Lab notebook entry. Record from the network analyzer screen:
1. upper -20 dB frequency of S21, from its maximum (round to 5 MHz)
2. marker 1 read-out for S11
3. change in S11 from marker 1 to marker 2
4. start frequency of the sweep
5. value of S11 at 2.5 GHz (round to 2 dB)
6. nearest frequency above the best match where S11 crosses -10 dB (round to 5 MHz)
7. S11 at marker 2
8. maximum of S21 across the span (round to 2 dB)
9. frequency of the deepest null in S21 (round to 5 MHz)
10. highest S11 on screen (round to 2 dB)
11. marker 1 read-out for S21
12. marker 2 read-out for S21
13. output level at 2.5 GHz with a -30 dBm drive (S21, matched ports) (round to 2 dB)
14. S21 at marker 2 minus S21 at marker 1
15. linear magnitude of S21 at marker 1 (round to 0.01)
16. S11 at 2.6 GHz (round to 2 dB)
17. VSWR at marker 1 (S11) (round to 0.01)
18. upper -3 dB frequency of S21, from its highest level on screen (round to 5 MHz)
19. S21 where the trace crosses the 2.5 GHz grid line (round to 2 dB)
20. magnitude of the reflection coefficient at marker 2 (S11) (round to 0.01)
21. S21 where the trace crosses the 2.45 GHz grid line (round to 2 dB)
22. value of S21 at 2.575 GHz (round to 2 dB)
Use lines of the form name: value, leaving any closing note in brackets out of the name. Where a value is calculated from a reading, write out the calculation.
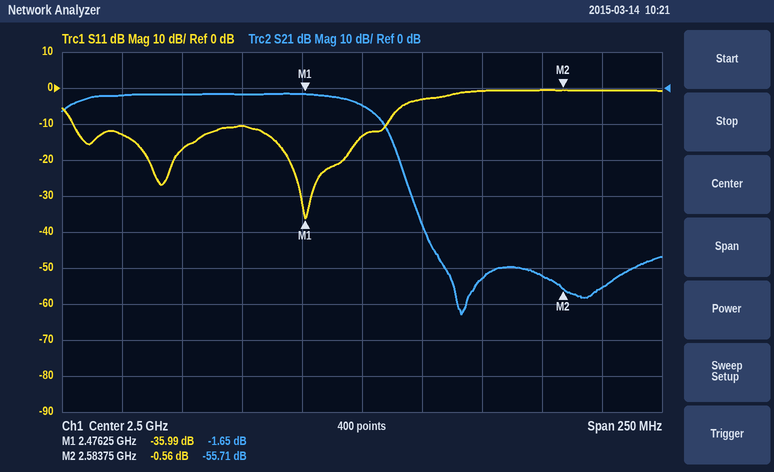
upper -20 dB frequency of S21, from its maximum: 2.515 GHz
marker 1 read-out for S11: -35.99 dB
change in S11 from marker 1 to marker 2: -0.56 − (-35.99) = 35.43 dB
start frequency of the sweep: 2.375 GHz
value of S11 at 2.5 GHz: -14 dB
nearest frequency above the best match where S11 crosses -10 dB: 2.510 GHz
S11 at marker 2: -0.56 dB
maximum of S21 across the span: -2 dB
frequency of the deepest null in S21: 2.540 GHz
highest S11 on screen: 0 dB
marker 1 read-out for S21: -1.65 dB
marker 2 read-out for S21: -55.71 dB
output level at 2.5 GHz with a -30 dBm drive (S21, matched ports): -30 dBm + (-4 dB) = -34 dBm
S21 at marker 2 minus S21 at marker 1: -55.71 − (-1.65) = -54.06 dB
linear magnitude of S21 at marker 1: 10^(-1.65/20) ≈ 0.83
S11 at 2.6 GHz: 0 dB
VSWR at marker 1 (S11): (1 + 0.0159)/(1 − 0.0159) ≈ 1.03
upper -3 dB frequency of S21, from its highest level on screen: 2.500 GHz
S21 where the trace crosses the 2.5 GHz grid line: -4 dB
magnitude of the reflection coefficient at marker 2 (S11): 10^(-0.56/20) ≈ 0.94
S21 where the trace crosses the 2.45 GHz grid line: -2 dB
value of S21 at 2.575 GHz: -52 dB
